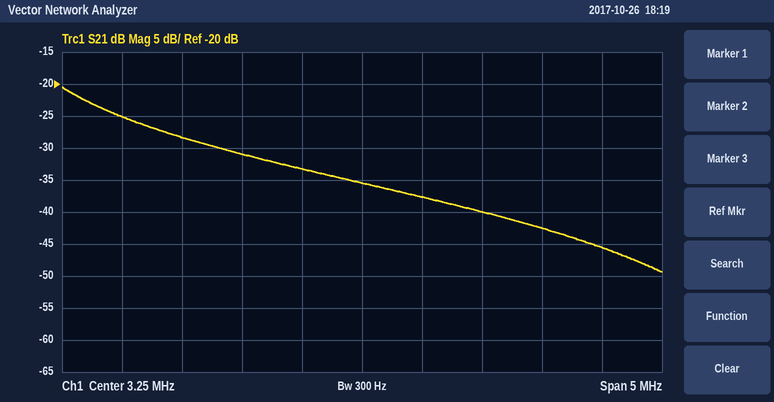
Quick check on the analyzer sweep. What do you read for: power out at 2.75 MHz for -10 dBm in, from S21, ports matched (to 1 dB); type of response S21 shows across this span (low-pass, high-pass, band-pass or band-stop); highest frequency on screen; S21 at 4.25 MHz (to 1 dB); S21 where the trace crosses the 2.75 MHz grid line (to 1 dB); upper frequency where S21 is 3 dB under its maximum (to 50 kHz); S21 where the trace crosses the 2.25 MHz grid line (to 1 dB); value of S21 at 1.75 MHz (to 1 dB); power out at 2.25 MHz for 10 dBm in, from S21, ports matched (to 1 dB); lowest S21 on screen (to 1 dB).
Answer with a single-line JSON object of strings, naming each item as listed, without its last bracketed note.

{"power out at 2.75 MHz for -10 dBm in, from S21, ports matched": "-43 dBm", "type of response S21 shows across this span": "low-pass", "highest frequency on screen": "5.75 MHz", "S21 at 4.25 MHz": "-40 dB", "S21 where the trace crosses the 2.75 MHz grid line": "-33 dB", "upper frequency where S21 is 3 dB under its maximum": "1.05 MHz", "S21 where the trace crosses the 2.25 MHz grid line": "-31 dB", "value of S21 at 1.75 MHz": "-28 dB", "power out at 2.25 MHz for 10 dBm in, from S21, ports matched": "-21 dBm", "lowest S21 on screen": "-49 dB"}
